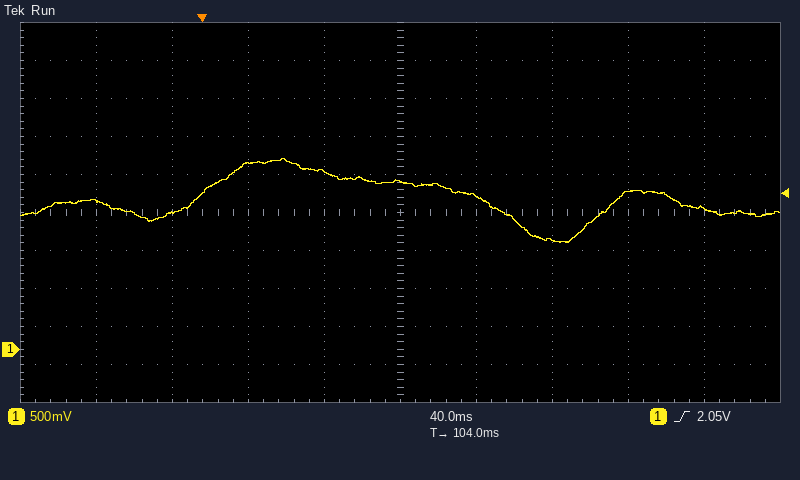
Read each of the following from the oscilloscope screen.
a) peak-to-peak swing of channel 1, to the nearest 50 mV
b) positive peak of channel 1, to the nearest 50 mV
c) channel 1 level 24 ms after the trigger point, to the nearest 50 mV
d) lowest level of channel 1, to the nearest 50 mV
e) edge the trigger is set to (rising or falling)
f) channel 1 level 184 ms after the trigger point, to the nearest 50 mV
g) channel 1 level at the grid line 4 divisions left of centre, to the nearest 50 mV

1.10 V
2.50 V
2.45 V
1.40 V
rising
1.45 V
1.95 V
